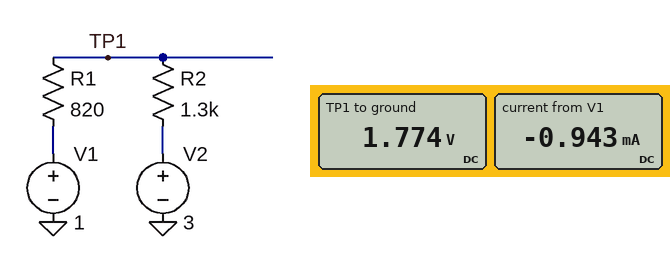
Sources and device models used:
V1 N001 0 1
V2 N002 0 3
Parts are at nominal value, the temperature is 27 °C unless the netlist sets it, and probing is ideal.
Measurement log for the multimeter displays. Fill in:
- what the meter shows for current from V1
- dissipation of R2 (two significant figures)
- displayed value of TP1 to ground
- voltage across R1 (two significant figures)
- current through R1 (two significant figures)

-0.943 mA
1.2 mW
1.774 V
770 mV
940 µA
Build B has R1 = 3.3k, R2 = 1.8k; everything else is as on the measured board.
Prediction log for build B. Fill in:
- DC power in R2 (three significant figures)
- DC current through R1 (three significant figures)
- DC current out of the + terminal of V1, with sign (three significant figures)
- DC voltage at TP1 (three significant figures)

277 µW
392 µA
-392 µA
2.29 V
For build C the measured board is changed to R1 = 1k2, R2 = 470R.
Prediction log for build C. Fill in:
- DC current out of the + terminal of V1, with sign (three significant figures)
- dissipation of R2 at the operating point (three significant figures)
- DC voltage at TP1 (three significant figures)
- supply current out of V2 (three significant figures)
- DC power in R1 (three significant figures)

-1.20 mA
674 µW
2.44 V
1.20 mA
1.72 mW
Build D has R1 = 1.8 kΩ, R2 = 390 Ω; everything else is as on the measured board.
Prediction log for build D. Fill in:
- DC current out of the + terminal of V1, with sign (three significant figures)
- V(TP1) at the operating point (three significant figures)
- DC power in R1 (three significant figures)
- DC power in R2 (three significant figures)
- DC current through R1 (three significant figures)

-913 µA
2.64 V
1.50 mW
325 µW
913 µA
